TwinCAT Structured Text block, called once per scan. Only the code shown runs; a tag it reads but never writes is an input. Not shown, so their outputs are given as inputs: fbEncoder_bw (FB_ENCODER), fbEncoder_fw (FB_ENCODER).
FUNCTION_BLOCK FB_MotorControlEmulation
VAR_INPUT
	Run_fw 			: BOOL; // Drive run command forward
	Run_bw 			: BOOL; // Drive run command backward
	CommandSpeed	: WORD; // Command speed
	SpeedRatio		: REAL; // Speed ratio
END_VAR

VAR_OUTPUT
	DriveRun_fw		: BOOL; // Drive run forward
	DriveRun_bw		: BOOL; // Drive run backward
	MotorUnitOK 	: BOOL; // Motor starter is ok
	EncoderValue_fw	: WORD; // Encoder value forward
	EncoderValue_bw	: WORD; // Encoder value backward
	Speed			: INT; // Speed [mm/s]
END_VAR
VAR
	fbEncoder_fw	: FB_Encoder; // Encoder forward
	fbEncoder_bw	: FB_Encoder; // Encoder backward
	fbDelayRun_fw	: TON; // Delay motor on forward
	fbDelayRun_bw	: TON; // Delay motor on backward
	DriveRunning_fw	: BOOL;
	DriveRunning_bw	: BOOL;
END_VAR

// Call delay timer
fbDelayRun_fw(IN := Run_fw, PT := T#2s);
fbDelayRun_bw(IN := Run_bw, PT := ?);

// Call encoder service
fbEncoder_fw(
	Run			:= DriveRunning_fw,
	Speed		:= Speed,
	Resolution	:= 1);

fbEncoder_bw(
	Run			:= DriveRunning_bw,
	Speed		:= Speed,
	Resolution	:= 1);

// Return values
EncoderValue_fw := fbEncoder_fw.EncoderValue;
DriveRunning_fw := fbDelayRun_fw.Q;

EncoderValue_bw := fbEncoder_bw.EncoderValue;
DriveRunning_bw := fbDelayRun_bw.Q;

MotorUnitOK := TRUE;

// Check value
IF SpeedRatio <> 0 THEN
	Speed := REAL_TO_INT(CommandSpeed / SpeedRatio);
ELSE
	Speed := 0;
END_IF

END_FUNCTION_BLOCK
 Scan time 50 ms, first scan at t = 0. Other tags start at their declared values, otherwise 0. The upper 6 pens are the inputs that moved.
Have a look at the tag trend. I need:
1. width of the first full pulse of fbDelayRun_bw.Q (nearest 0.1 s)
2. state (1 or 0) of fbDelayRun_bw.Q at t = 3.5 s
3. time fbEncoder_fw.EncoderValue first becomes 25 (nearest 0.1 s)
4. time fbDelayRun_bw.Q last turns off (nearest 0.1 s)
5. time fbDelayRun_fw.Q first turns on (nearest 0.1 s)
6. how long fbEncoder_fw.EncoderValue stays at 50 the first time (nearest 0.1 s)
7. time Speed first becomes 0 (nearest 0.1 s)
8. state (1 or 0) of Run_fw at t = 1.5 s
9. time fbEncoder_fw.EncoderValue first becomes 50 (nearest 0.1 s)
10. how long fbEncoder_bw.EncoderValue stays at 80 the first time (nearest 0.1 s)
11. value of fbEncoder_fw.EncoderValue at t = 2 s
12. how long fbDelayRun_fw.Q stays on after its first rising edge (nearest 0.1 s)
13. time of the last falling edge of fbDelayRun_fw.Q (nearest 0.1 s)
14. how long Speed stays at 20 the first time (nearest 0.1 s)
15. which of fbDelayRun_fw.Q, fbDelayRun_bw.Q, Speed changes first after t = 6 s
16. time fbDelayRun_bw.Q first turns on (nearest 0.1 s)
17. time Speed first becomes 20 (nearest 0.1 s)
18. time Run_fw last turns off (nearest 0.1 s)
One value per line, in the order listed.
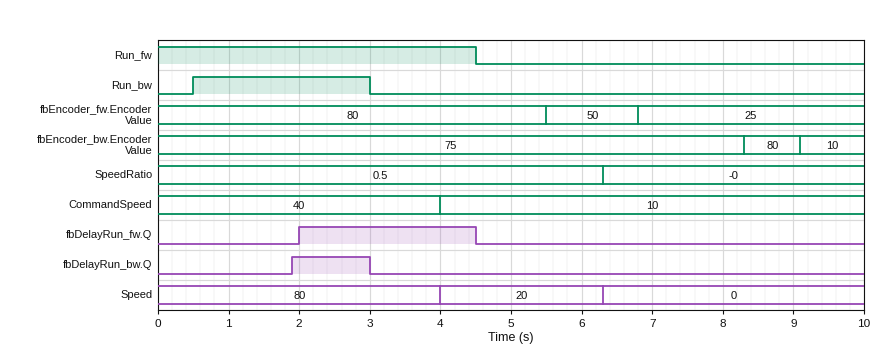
1.1 s
0
6.8 s
3.0 s
2.0 s
1.3 s
6.3 s
1
5.5 s
0.8 s
80
2.5 s
4.5 s
2.3 s
Speed
1.9 s
4.0 s
4.5 s
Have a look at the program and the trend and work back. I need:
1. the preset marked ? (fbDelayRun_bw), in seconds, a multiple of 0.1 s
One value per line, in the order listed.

1.4 s
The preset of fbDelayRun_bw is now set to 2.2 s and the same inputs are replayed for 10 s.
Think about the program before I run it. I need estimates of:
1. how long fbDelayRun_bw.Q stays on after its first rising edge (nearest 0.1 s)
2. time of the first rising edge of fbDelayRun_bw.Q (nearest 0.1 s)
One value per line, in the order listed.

0.3 s
2.7 s
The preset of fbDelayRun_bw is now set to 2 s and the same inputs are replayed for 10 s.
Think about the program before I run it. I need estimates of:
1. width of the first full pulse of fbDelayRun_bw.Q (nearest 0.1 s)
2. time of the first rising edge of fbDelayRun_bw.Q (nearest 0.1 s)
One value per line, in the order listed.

0.5 s
2.5 s
